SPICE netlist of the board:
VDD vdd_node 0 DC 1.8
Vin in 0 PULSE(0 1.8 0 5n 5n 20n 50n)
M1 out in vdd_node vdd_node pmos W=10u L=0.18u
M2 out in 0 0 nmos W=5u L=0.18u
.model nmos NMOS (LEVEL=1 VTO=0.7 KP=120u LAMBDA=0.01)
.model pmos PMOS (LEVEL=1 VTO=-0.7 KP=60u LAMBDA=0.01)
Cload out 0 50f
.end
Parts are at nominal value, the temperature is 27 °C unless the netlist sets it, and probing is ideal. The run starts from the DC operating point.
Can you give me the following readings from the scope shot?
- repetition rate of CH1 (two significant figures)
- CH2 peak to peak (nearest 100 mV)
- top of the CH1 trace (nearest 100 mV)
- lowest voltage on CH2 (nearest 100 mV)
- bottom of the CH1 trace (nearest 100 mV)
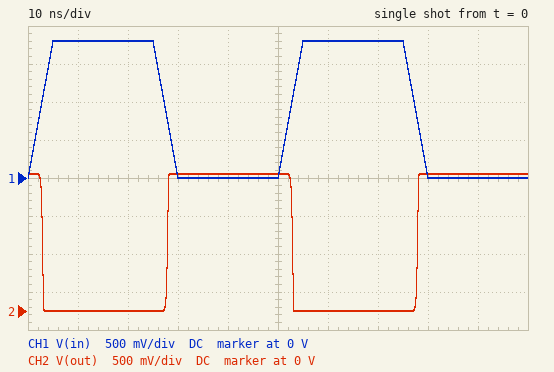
20 MHz
1.8 V
1.8 V
0 V
0 V
